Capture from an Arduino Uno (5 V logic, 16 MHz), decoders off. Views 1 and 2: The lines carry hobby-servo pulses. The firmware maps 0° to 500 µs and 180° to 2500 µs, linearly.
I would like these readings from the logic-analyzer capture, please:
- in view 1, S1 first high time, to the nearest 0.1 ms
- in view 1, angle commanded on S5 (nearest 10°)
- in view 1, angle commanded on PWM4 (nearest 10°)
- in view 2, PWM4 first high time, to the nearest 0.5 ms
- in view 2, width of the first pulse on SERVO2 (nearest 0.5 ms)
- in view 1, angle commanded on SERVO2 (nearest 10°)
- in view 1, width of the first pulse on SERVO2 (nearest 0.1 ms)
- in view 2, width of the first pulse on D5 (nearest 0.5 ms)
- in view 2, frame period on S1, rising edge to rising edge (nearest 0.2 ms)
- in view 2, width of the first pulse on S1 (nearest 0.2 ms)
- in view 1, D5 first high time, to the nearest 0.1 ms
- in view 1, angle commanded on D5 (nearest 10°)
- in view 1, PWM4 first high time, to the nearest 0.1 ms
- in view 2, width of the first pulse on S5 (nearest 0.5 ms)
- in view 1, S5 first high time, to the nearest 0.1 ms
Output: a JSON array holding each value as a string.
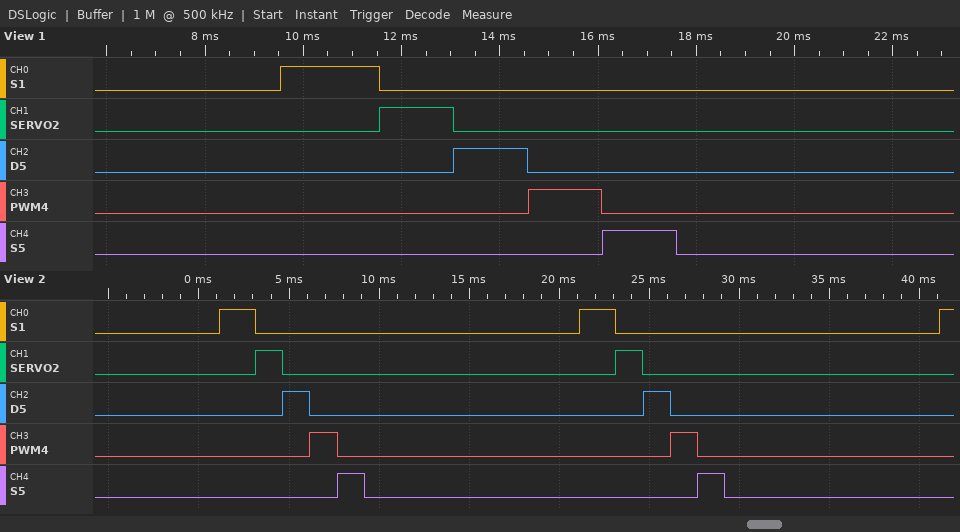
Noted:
["2.0 ms", "90°", "90°", "1.5 ms", "1.5 ms", "90°", "1.5 ms", "1.5 ms", "20.0 ms", "2.0 ms", "1.5 ms", "90°", "1.5 ms", "1.5 ms", "1.5 ms"]
